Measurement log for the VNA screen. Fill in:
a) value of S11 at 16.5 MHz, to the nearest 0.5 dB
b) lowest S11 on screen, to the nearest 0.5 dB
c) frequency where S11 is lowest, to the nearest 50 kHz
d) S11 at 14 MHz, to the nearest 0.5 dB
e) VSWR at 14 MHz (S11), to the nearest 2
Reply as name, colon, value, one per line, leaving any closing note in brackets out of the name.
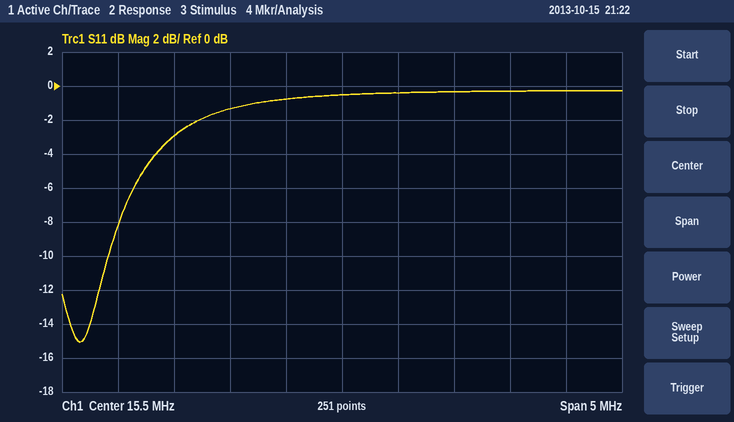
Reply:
value of S11 at 16.5 MHz, to the nearest 0.5 dB: -0.5 dB
lowest S11 on screen, to the nearest 0.5 dB: -15.0 dB
frequency where S11 is lowest, to the nearest 50 kHz: 13.15 MHz
S11 at 14 MHz, to the nearest 0.5 dB: -3.0 dB
VSWR at 14 MHz (S11), to the nearest 2: 6
